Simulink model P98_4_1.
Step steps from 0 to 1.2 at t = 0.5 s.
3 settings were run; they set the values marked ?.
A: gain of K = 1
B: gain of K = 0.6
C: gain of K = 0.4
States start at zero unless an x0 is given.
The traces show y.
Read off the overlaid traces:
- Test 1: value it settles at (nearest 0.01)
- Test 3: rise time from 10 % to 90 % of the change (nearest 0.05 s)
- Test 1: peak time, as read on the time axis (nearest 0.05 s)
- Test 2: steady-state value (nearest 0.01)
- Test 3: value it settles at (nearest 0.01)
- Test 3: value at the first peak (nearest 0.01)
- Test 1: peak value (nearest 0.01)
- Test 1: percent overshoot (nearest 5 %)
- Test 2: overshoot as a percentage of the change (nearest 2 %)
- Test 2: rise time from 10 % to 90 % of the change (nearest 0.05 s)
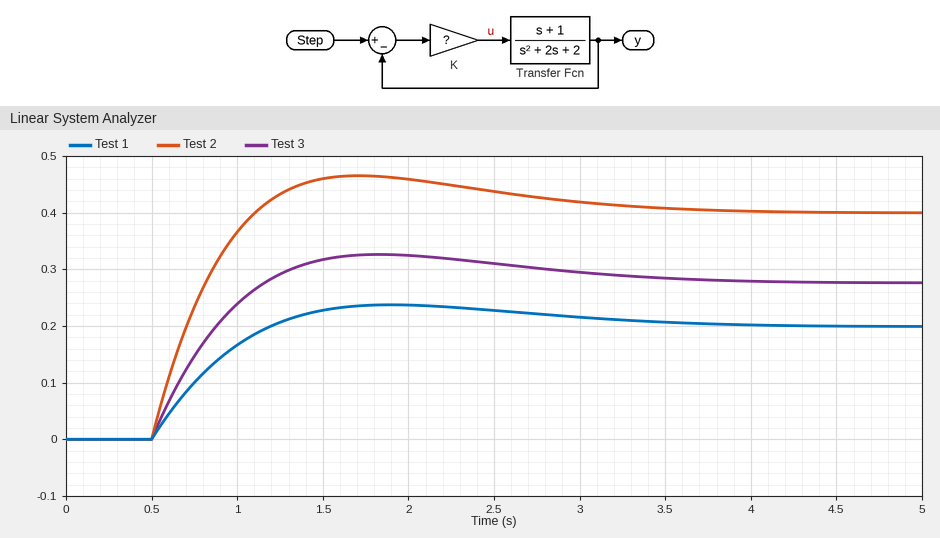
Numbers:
0.20
0.50 s
1.90 s
0.40
0.28
0.33
0.24
20 %
16 %
0.45 s
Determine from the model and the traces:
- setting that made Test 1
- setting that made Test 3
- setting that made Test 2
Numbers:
C
B
A
